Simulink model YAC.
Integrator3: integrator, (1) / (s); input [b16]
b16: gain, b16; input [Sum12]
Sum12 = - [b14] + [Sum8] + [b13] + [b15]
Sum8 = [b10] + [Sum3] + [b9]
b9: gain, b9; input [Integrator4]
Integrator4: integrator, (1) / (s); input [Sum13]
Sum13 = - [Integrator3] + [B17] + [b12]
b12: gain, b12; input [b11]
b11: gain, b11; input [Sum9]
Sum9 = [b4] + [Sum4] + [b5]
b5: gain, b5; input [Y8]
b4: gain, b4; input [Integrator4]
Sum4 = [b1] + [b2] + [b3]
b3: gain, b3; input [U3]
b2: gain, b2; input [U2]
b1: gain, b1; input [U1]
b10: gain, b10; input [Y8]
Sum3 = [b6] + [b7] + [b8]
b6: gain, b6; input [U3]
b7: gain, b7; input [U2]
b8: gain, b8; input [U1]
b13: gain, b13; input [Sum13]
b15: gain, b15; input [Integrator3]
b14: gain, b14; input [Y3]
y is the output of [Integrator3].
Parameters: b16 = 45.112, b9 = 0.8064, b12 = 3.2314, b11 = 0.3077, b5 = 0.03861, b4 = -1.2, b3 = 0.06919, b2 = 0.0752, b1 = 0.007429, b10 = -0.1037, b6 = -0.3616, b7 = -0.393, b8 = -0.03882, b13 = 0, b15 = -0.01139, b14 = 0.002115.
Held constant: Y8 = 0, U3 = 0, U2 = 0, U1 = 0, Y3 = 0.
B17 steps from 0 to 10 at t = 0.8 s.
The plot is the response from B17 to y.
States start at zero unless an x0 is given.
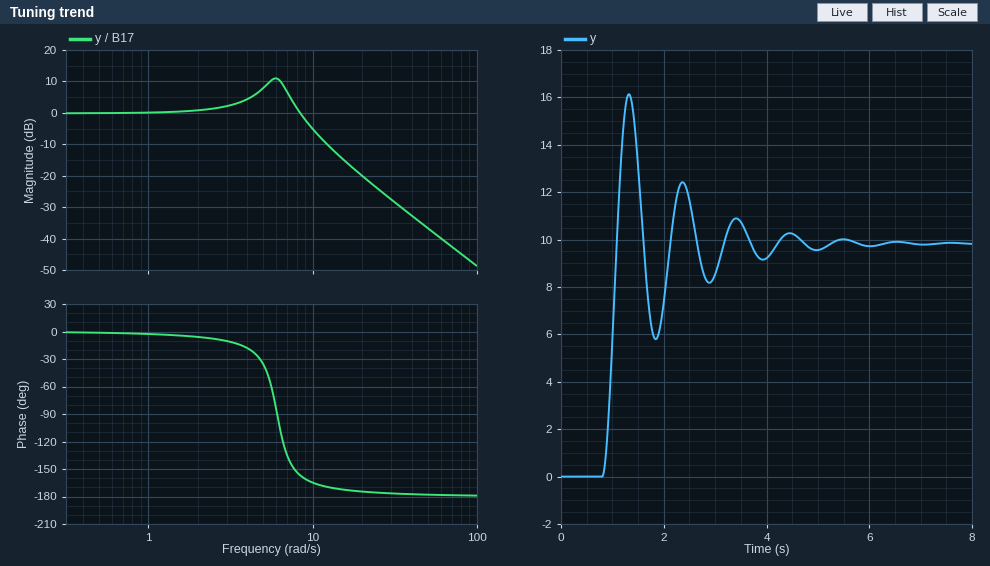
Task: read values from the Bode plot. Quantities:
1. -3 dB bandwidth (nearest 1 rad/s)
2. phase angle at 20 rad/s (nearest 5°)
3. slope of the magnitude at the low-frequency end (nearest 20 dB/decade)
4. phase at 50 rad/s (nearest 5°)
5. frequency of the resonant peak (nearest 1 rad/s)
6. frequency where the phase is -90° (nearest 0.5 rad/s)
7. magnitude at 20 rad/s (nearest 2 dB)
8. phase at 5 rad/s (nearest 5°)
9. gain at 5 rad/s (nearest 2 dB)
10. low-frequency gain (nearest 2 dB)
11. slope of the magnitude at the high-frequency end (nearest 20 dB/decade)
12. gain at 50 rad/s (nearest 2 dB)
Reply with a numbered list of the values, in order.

1. 9 rad/s
2. -175°
3. 0 dB/decade
4. -180°
5. 6 rad/s
6. 6.0 rad/s
7. -20 dB
8. -35°
9. 8 dB
10. 0 dB
11. -40 dB/decade
12. -36 dB
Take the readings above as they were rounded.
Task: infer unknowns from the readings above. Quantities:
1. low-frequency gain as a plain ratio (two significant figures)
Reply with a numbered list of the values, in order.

1. 1.0
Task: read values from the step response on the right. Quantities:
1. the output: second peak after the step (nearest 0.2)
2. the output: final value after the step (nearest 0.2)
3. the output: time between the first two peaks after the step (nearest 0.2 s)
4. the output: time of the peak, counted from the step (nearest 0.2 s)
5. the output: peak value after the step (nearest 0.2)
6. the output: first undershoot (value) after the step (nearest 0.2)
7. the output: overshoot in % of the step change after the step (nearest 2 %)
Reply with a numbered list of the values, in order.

1. 12.4
2. 9.8
3. 1.0 s
4. 0.6 s
5. 16.2
6. 5.8
7. 64 %
